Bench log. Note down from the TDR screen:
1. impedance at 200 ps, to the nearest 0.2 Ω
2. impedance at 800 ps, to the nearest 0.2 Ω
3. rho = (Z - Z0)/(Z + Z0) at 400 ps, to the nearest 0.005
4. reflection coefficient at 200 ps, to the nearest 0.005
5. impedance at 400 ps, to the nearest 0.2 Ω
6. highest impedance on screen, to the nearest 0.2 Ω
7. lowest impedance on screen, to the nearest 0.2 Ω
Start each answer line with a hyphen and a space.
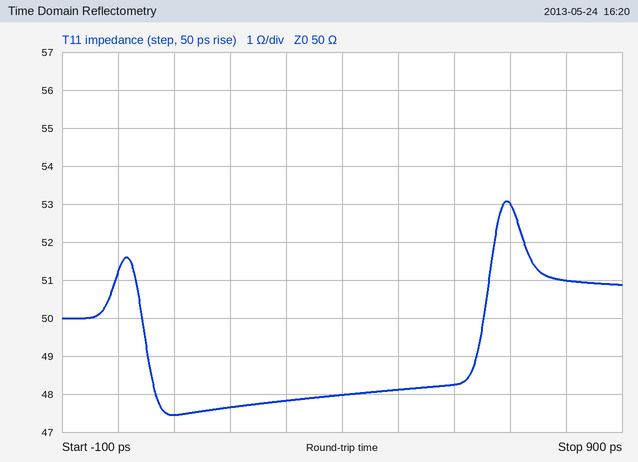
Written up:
- 47.6 Ω
- 51.0 Ω
- -0.020
- -0.025
- 48.0 Ω
- 53.0 Ω
- 47.4 Ω
